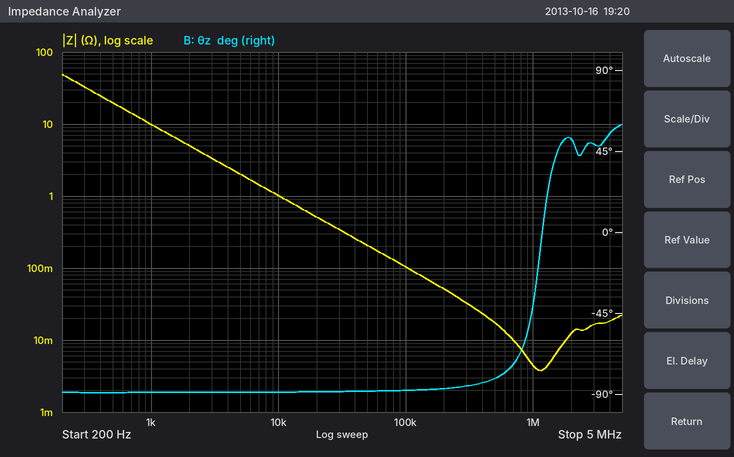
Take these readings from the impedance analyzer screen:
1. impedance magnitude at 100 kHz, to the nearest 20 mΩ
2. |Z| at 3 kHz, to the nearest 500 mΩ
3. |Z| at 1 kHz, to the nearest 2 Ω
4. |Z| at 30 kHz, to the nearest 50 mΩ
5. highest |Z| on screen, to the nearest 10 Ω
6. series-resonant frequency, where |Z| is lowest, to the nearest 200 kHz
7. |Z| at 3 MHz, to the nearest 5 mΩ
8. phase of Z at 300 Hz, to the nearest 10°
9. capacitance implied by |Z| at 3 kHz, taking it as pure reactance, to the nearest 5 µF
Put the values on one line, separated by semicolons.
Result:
100 mΩ; 3.5 Ω; 10 Ω; 350 mΩ; 50 Ω; 1.2 MHz; 15 mΩ; -90°; 15 µF
